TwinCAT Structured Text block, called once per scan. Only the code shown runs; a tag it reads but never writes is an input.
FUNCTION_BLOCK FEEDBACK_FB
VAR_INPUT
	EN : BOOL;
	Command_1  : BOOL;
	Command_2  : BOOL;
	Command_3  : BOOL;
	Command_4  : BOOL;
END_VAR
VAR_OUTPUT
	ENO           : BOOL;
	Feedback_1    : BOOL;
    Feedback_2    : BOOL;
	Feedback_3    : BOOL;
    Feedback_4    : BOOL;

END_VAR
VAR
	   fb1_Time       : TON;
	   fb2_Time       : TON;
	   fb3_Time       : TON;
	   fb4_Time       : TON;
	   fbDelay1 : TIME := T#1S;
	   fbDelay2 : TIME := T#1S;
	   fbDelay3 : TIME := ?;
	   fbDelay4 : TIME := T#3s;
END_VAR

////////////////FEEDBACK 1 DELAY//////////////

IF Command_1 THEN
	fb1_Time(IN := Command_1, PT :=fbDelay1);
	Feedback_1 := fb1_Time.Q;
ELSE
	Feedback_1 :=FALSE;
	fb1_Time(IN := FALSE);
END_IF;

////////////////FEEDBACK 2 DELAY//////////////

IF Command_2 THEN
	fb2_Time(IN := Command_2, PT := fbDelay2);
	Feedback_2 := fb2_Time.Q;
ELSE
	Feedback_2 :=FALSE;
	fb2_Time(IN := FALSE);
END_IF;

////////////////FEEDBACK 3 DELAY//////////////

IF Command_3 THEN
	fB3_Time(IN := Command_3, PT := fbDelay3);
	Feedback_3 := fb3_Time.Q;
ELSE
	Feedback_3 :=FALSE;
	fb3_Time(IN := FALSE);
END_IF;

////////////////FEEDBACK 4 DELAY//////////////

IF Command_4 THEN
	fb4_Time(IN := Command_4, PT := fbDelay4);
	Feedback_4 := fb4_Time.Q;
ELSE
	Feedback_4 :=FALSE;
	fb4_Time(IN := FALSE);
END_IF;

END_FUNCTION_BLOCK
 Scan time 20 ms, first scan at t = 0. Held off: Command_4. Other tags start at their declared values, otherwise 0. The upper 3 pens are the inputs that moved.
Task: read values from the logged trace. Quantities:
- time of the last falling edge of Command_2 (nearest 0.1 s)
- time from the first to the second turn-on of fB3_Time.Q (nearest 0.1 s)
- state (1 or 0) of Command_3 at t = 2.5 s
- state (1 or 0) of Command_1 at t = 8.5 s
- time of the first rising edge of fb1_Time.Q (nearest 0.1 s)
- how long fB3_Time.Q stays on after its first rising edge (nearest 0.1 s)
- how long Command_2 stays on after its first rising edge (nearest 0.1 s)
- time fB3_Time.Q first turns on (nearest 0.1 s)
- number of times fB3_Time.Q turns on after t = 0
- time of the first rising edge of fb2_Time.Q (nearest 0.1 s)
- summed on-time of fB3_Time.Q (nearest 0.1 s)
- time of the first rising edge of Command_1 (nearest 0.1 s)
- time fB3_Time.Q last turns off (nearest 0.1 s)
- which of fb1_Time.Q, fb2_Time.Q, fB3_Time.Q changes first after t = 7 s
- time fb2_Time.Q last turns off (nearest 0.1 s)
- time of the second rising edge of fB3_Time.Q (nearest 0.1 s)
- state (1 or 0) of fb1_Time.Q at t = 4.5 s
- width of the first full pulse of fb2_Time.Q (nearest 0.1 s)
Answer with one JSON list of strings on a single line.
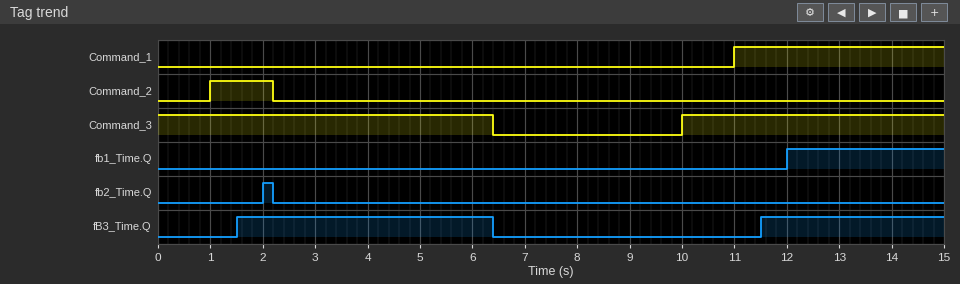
["2.2 s", "10.0 s", "1", "0", "12.0 s", "4.9 s", "1.2 s", "1.5 s", "2", "2.0 s", "8.4 s", "11.0 s", "6.4 s", "fB3_Time.Q", "2.2 s", "11.5 s", "0", "0.2 s"]
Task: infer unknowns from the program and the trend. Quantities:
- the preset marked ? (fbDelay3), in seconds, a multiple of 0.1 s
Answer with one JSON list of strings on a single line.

["1.5 s"]
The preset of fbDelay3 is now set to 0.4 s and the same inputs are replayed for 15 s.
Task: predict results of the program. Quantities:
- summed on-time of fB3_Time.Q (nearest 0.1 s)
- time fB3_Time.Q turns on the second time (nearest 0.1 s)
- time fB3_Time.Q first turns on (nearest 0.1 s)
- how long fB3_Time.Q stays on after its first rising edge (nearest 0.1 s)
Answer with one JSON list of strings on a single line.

["10.6 s", "10.4 s", "0.4 s", "6.0 s"]
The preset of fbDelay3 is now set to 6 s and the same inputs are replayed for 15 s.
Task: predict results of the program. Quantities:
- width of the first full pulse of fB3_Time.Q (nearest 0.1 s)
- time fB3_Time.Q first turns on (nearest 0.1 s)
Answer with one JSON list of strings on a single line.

["0.4 s", "6.0 s"]
